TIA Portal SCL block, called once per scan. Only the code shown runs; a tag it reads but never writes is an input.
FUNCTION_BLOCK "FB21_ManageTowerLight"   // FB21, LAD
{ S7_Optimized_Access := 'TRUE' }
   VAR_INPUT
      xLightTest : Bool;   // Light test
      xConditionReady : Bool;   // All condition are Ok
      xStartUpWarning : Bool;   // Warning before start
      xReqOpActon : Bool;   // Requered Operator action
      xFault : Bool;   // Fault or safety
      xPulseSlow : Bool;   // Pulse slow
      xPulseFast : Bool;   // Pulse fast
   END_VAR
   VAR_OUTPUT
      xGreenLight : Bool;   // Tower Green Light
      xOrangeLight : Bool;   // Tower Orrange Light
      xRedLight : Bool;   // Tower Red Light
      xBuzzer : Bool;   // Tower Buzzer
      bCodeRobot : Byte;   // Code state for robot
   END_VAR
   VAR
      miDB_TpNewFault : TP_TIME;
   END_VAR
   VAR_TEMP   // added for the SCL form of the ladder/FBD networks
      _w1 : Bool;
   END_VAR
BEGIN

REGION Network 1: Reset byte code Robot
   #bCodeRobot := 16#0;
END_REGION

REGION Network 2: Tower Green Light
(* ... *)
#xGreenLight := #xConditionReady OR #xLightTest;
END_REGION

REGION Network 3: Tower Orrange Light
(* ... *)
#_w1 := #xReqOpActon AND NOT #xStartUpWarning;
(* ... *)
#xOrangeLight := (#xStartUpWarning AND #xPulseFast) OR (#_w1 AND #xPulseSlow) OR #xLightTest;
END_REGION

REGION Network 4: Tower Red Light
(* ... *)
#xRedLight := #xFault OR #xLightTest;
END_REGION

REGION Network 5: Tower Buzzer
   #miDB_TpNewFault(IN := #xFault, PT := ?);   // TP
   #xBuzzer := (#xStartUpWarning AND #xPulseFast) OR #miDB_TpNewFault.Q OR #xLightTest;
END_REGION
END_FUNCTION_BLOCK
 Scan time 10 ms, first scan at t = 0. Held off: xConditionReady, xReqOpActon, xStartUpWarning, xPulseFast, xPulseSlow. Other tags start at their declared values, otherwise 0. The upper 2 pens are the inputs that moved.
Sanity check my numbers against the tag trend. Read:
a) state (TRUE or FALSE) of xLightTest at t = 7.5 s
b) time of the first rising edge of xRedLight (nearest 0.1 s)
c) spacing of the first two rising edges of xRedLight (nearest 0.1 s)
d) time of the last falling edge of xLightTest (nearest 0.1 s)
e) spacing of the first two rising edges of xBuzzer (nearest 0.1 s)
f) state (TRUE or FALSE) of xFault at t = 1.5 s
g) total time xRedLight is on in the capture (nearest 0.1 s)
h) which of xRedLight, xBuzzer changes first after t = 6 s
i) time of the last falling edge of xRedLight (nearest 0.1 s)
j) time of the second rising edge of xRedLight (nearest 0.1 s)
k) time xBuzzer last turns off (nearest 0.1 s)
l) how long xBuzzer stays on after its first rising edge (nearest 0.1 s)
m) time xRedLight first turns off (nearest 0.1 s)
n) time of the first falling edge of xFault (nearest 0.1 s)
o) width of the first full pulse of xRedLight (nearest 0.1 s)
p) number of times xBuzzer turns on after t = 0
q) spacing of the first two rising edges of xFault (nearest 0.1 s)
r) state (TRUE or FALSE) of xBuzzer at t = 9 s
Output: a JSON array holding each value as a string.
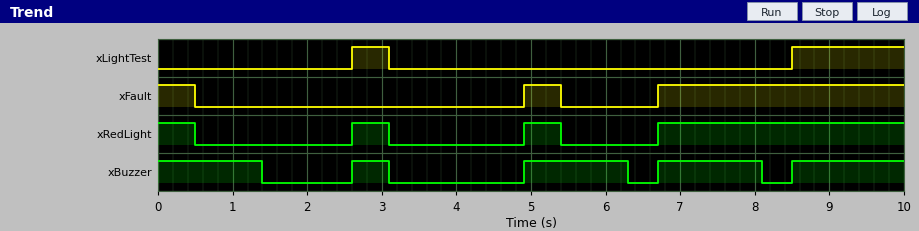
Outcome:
["FALSE", "2.6 s", "2.3 s", "3.1 s", "2.3 s", "FALSE", "4.8 s", "xBuzzer", "5.4 s", "4.9 s", "8.1 s", "0.5 s", "0.5 s", "0.5 s", "0.5 s", "4", "1.8 s", "TRUE"]
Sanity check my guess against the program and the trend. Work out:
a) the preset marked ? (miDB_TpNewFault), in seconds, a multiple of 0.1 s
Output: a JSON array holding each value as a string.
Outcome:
["1.4 s"]
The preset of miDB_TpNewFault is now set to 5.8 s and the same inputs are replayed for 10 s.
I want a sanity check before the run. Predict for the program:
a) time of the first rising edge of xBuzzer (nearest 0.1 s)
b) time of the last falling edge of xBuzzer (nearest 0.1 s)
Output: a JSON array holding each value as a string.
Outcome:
["6.7 s", "5.8 s"]
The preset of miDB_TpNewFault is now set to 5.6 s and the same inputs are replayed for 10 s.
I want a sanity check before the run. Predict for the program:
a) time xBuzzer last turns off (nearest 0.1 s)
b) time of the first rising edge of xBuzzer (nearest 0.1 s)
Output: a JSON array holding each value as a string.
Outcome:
["5.6 s", "6.7 s"]
